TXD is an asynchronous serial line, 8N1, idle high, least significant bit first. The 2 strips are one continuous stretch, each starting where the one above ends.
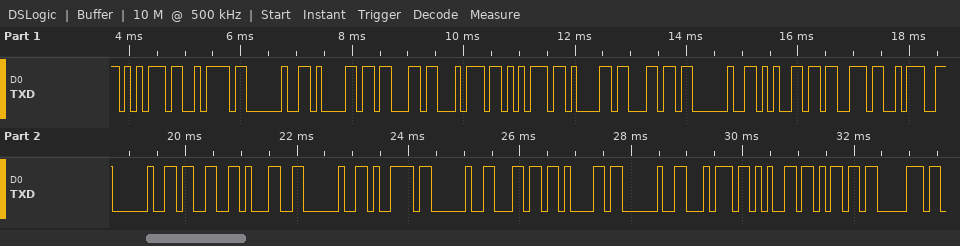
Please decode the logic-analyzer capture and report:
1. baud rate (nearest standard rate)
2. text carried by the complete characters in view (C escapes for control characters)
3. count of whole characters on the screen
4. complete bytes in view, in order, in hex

9600 baud
"uz actual es: 31 y la temp"
26
75 7A 20 61 63 74 75 61 6C 20 65 73 3A 20 33 31 20 79 20 6C 61 20 74 65 6D 70
